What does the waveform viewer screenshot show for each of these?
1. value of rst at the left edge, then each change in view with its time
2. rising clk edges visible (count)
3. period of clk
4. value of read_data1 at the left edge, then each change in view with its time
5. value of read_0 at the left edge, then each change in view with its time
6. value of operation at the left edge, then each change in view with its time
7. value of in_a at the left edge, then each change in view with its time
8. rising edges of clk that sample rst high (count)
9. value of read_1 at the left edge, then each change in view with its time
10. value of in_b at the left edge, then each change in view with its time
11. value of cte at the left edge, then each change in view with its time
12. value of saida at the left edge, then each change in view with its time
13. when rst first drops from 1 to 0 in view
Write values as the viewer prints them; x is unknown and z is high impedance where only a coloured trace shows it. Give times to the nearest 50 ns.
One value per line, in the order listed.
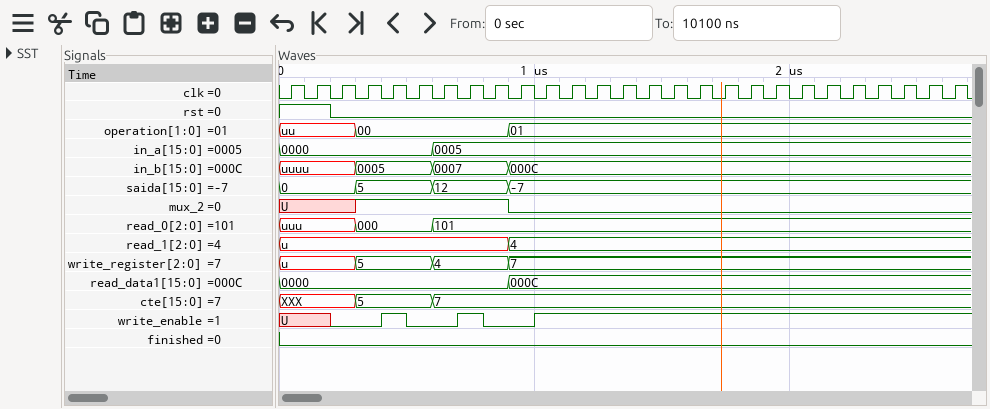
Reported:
1, 0 at 200 ns
27
100 ns
0000, 000C at 900 ns
uuu, 000 at 300 ns, 101 at 600 ns
uu, 00 at 300 ns, 01 at 900 ns
0000, 0005 at 600 ns
2
u, 4 at 900 ns
uuuu, 0005 at 300 ns, 0007 at 600 ns, 000C at 900 ns
XXX, 5 at 300 ns, 7 at 600 ns
0, 5 at 300 ns, 12 at 600 ns, -7 at 900 ns
200 ns
